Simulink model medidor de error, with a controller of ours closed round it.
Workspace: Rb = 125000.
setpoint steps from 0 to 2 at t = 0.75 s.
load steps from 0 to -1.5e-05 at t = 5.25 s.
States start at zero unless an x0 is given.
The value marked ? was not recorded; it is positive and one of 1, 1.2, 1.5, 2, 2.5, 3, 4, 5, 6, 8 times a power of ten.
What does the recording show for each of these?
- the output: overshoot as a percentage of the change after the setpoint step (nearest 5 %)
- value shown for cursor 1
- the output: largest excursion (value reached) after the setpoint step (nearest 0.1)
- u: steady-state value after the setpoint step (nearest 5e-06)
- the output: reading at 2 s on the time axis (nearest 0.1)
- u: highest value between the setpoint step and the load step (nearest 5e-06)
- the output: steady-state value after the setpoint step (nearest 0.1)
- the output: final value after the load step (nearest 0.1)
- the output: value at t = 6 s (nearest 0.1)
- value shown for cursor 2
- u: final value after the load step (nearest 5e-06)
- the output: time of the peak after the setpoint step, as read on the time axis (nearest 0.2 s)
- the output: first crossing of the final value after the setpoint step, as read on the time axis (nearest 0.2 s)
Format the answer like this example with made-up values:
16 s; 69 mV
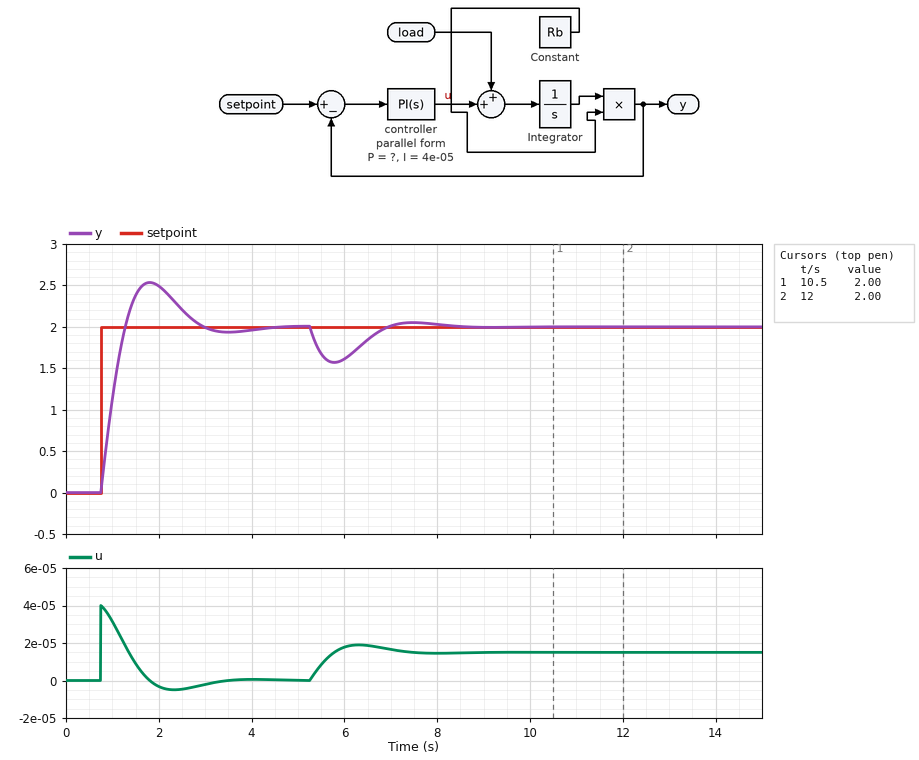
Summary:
25 %; 2.00; 2.5; 0.000000; 2.5; 0.000040; 2.0; 2.0; 1.6; 2.00; 0.000015; 1.8 s; 1.2 s
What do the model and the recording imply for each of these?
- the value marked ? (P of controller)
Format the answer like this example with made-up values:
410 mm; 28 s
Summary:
2e-05
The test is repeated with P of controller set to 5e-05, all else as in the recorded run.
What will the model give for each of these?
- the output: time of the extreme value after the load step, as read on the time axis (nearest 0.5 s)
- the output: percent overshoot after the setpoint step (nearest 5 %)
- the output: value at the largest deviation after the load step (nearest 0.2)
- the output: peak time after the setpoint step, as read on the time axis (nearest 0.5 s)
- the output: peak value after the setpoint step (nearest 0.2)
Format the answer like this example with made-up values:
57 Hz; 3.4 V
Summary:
5.5 s; 10 %; 1.8; 1.5 s; 2.2
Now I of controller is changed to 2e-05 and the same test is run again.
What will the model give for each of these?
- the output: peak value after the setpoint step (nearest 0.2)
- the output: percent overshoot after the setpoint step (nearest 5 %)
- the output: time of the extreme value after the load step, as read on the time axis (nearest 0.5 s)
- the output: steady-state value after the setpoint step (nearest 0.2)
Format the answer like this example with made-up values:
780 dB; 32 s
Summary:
2.4; 20 %; 6.0 s; 2.0
